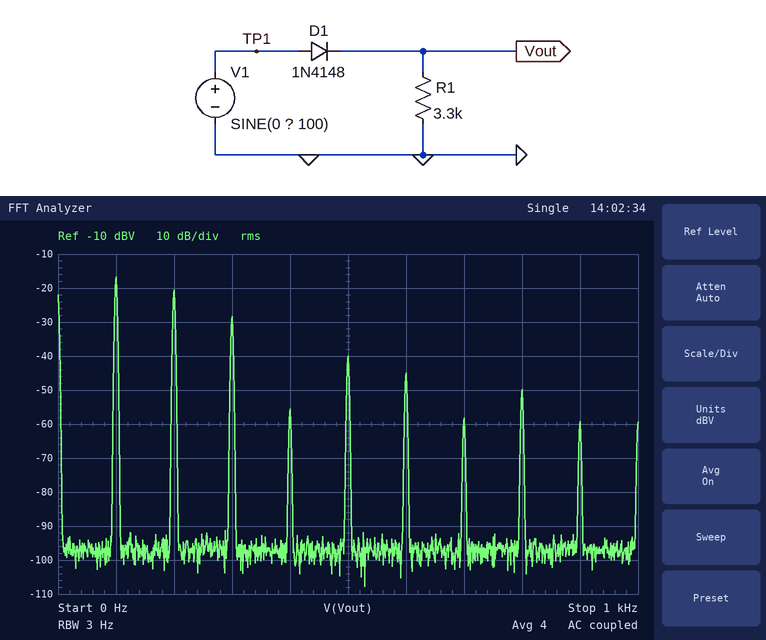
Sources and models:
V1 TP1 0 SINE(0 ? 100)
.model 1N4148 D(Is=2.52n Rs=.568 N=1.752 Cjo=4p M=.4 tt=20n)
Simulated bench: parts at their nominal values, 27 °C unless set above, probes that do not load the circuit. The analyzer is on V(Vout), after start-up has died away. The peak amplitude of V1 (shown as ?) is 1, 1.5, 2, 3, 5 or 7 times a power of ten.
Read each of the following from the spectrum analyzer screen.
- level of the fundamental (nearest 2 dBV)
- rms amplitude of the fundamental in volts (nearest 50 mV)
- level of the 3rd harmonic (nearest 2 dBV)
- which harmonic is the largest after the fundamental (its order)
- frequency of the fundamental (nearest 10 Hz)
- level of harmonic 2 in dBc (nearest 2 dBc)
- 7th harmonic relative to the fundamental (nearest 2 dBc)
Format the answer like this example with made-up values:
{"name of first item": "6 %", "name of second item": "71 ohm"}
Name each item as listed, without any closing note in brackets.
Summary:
{"level of the fundamental": "-16 dBV", "rms amplitude of the fundamental in volts": "150 mV", "level of the 3rd harmonic": "-28 dBV", "which harmonic is the largest after the fundamental": "2", "frequency of the fundamental": "100 Hz", "level of harmonic 2 in dBc": "-4 dBc", "7th harmonic relative to the fundamental": "-42 dBc"}
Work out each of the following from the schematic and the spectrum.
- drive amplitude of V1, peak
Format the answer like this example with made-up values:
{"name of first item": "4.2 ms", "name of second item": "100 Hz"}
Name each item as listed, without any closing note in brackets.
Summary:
{"drive amplitude of V1, peak": "1 V"}
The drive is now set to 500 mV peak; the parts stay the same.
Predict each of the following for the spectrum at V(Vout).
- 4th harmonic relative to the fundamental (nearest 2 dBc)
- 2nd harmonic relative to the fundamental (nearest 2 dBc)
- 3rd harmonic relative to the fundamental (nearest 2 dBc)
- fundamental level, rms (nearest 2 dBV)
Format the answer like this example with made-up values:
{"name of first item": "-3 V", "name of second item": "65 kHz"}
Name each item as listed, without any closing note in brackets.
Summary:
{"4th harmonic relative to the fundamental": "-12 dBc", "2nd harmonic relative to the fundamental": "-2 dBc", "3rd harmonic relative to the fundamental": "-6 dBc", "fundamental level, rms": "-34 dBV"}
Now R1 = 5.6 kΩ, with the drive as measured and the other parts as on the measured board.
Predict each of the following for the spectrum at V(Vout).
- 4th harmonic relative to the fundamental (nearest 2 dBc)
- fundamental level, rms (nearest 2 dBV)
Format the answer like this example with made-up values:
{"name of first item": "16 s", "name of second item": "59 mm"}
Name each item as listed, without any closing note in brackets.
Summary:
{"4th harmonic relative to the fundamental": "-58 dBc", "fundamental level, rms": "-16 dBV"}
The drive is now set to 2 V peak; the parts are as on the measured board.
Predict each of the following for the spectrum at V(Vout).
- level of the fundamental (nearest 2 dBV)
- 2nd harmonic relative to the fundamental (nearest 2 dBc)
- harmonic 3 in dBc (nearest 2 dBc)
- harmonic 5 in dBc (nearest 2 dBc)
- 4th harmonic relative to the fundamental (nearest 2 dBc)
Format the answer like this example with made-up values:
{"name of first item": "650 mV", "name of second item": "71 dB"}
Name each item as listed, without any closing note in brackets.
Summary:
{"level of the fundamental": "-6 dBV", "2nd harmonic relative to the fundamental": "-6 dBc", "harmonic 3 in dBc": "-18 dBc", "harmonic 5 in dBc": "-24 dBc", "4th harmonic relative to the fundamental": "-24 dBc"}
